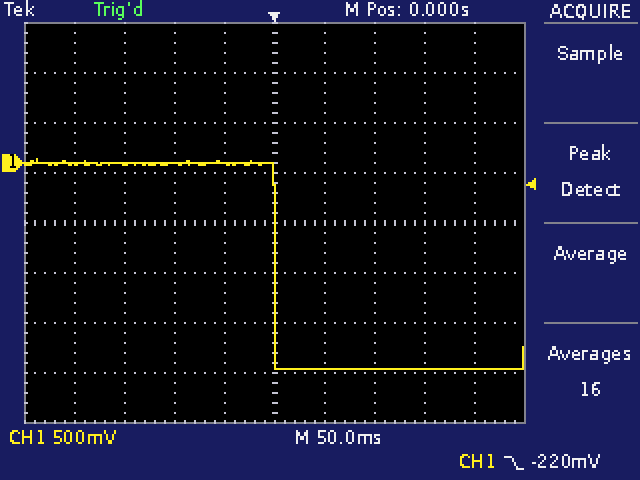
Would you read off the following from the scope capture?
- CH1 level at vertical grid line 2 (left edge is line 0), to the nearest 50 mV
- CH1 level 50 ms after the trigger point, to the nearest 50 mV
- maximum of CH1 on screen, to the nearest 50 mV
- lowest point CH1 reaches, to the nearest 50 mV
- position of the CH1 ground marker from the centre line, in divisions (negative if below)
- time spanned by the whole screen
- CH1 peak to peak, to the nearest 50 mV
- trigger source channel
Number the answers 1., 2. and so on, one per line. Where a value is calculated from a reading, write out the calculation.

1. 0 mV
2. -2.05 V
3. 50 mV
4. -2.05 V
5. +1.2 div
6. 500 ms
7. 50 mV − (-2.05 V) = 2.10 V
8. CH1
